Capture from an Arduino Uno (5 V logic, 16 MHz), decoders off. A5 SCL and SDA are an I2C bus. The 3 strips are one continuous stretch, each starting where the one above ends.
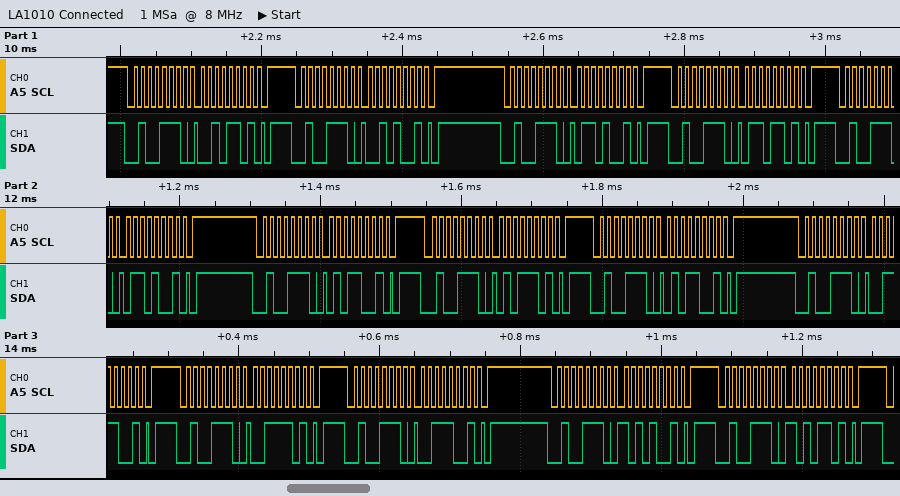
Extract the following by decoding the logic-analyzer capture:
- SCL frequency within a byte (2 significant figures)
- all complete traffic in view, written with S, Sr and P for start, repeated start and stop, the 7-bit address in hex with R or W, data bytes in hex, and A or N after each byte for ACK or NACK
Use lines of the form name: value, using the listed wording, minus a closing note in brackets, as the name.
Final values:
SCL frequency within a byte: 100 kHz
all complete traffic in view, written with S, Sr and P for start, repeated start and stop, the 7-bit address in hex with R or W, data bytes in hex, and A or N after each byte for ACK or NACK: S 27W A 2D A P S 27W A 29 A P S 27W A 69 A P S 27W A 6D A P S 27W A 69 A P S 27W A 59 A P S 27W A 5D A P S 27W A 59 A P S 27W A 39 A P S 27W A 3D A P S 27W A 39 A P S 27W A A9 A P S 27W A AD A P
